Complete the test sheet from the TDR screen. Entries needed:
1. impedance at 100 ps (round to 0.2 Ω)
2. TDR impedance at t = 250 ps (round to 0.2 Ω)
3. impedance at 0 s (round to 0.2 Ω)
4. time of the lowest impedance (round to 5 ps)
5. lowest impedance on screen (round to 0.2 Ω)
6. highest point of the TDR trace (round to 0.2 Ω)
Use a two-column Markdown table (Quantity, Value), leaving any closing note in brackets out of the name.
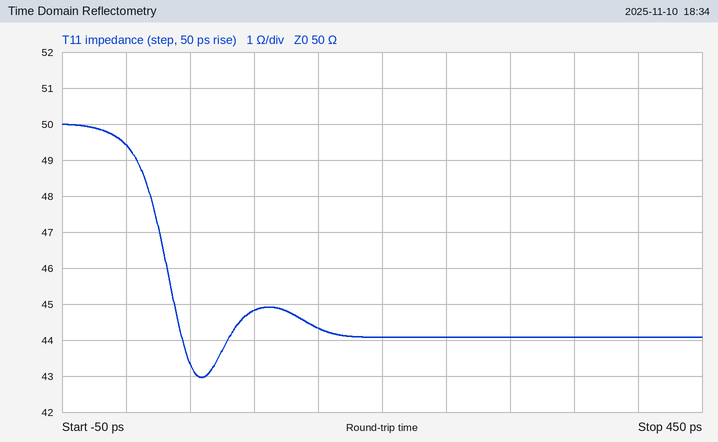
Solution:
| Quantity | Value |
|---|---|
| impedance at 100 ps | 44.8 Ω |
| TDR impedance at t = 250 ps | 44.0 Ω |
| impedance at 0 s | 49.4 Ω |
| time of the lowest impedance | 60 ps |
| lowest impedance on screen | 43.0 Ω |
| highest point of the TDR trace | 50.0 Ω |
